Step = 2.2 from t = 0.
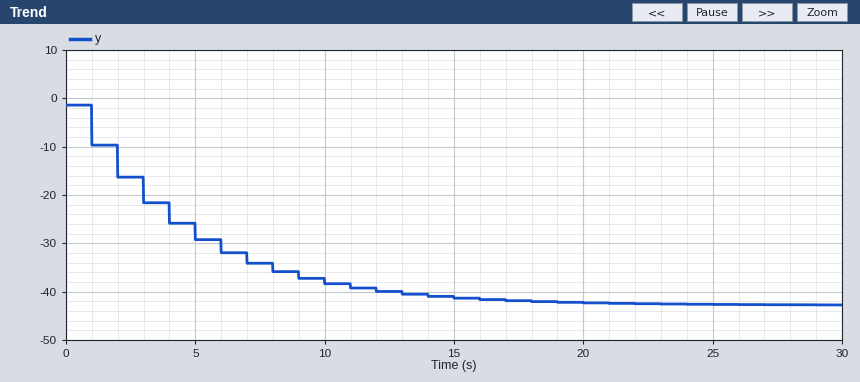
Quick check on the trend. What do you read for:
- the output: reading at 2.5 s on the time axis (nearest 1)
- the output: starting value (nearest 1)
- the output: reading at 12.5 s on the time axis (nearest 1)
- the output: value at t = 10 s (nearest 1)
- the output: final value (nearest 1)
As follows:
-16
-1
-40
-38
-43
